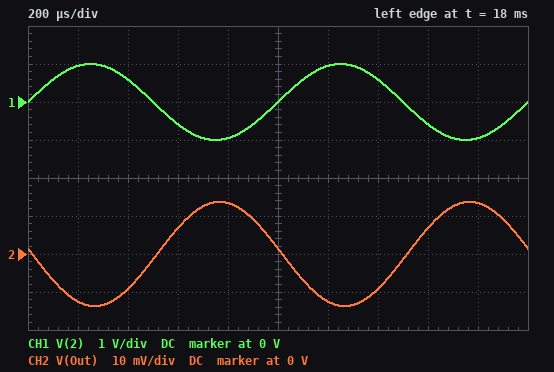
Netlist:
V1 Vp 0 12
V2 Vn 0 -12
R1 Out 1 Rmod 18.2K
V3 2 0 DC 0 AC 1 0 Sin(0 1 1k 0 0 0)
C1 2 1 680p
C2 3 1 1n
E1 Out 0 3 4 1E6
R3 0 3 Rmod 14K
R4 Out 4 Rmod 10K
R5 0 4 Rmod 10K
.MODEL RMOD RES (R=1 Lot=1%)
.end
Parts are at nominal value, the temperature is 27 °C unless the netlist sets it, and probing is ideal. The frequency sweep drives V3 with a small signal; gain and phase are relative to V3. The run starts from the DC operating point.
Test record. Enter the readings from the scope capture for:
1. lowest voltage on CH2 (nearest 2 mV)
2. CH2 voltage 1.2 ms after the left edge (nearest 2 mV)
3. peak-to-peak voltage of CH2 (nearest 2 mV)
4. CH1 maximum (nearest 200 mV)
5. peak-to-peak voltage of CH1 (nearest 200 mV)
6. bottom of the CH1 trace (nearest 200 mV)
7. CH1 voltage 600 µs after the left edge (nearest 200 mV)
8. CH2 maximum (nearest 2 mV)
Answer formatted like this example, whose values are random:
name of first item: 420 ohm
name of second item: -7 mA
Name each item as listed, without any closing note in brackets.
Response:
lowest voltage on CH2: -14 mV
CH2 voltage 1.2 ms after the left edge: -12 mV
peak-to-peak voltage of CH2: 28 mV
CH1 maximum: 1.0 V
peak-to-peak voltage of CH1: 2.0 V
bottom of the CH1 trace: -1.0 V
CH1 voltage 600 µs after the left edge: -600 mV
CH2 maximum: 14 mV
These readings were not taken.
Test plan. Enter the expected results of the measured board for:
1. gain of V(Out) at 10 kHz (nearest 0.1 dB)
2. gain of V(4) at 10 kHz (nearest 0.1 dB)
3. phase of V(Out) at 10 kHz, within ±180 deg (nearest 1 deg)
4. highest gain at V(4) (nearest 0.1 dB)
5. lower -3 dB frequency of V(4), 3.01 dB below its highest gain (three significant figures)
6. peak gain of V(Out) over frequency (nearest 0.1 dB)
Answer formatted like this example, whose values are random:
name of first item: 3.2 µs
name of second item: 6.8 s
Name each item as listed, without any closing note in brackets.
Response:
gain of V(Out) at 10 kHz: 2.0 dB
gain of V(4) at 10 kHz: -4.0 dB
phase of V(Out) at 10 kHz, within ±180 deg: 107 deg
highest gain at V(4): 0.2 dB
lower -3 dB frequency of V(4), 3.01 dB below its highest gain: 11.1 kHz
peak gain of V(Out) over frequency: 6.2 dB
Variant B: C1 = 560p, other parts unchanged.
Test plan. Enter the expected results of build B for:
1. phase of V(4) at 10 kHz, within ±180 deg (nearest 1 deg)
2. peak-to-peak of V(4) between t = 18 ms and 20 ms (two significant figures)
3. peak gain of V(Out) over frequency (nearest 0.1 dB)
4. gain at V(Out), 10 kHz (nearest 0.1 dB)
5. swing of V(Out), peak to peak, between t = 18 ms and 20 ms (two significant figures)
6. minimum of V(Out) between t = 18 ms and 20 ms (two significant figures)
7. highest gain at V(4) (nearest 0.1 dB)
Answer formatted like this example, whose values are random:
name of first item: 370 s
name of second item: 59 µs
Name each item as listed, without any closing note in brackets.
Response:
phase of V(4) at 10 kHz, within ±180 deg: 116 deg
peak-to-peak of V(4) between t = 18 ms and 20 ms: 11 mV
peak gain of V(Out) over frequency: 6.4 dB
gain at V(Out), 10 kHz: 1.0 dB
swing of V(Out), peak to peak, between t = 18 ms and 20 ms: 23 mV
minimum of V(Out) between t = 18 ms and 20 ms: -11 mV
highest gain at V(4): 0.3 dB
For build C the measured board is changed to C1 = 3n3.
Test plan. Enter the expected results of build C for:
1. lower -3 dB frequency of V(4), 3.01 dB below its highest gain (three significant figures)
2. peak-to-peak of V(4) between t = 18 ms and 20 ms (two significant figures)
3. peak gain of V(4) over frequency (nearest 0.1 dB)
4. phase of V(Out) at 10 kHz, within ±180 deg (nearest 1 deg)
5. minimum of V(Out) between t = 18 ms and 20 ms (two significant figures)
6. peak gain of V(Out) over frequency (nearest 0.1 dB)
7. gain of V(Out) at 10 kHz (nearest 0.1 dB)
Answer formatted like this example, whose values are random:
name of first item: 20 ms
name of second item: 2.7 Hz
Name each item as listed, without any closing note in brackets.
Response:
lower -3 dB frequency of V(4), 3.01 dB below its highest gain: 9.85 kHz
peak-to-peak of V(4) between t = 18 ms and 20 ms: 63 mV
peak gain of V(4) over frequency: 0 dB
phase of V(Out) at 10 kHz, within ±180 deg: 60 deg
minimum of V(Out) between t = 18 ms and 20 ms: -63 mV
peak gain of V(Out) over frequency: 6.0 dB
gain of V(Out) at 10 kHz: 3.1 dB
